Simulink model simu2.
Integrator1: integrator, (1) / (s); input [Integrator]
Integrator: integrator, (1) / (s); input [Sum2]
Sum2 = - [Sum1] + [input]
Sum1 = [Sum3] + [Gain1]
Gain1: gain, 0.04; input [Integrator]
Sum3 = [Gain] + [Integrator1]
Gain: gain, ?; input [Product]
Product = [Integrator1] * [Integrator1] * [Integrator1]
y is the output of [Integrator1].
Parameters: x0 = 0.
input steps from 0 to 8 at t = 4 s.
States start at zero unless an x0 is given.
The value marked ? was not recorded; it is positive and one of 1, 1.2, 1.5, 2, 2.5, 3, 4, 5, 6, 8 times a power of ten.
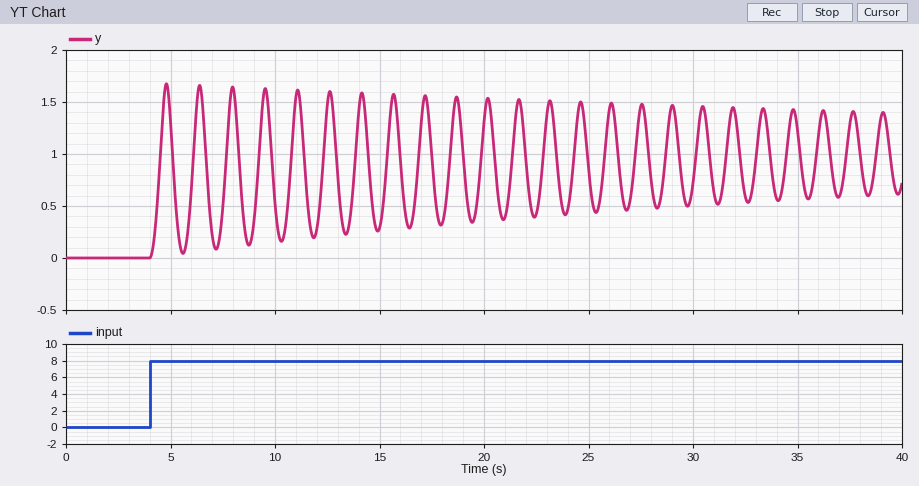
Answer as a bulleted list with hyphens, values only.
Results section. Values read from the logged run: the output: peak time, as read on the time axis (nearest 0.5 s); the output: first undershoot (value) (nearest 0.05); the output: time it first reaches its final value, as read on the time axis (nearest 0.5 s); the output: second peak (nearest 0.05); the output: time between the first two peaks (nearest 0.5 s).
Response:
- 5.0 s
- 0.05
- 4.5 s
- 1.65
- 1.5 s
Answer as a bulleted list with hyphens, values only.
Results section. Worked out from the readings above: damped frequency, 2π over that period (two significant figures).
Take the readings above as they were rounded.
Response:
- 4.2 rad/s
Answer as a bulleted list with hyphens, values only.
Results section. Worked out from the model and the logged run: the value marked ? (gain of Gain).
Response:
- 6
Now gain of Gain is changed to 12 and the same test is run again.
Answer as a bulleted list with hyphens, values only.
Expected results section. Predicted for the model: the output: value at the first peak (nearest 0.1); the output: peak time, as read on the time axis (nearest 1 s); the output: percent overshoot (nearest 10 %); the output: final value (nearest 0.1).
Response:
- 1.3
- 5 s
- 60 %
- 0.8
